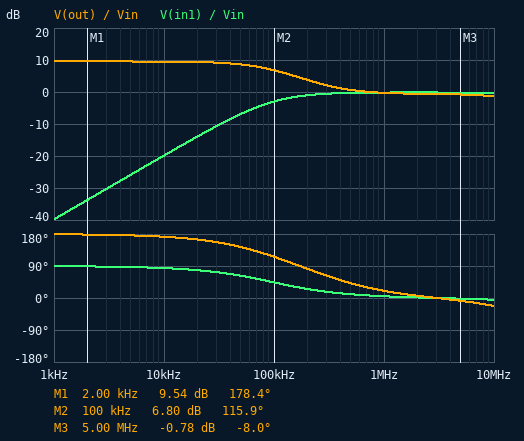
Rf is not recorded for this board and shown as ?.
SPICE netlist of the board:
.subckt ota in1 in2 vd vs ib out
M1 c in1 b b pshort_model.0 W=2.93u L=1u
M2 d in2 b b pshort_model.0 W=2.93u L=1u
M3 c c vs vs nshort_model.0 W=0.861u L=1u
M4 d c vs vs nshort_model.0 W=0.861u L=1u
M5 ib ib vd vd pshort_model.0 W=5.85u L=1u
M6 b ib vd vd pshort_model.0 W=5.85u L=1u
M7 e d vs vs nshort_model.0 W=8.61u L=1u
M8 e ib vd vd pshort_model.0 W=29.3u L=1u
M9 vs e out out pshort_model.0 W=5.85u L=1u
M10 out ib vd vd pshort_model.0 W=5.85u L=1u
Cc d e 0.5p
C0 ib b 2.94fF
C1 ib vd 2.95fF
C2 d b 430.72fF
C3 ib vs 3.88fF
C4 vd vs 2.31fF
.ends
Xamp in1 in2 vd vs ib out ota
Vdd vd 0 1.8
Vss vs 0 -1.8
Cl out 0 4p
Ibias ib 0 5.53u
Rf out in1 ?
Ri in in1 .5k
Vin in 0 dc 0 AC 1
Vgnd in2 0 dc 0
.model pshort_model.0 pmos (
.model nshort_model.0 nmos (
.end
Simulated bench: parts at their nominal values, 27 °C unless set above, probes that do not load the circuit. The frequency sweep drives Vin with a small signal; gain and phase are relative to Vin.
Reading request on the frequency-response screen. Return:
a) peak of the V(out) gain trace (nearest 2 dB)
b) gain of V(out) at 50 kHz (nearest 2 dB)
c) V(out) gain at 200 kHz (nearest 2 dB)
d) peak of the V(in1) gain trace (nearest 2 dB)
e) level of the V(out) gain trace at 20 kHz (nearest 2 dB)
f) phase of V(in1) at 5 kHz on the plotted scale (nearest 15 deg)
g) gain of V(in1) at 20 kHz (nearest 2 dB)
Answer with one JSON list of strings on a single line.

["10 dB", "8 dB", "4 dB", "0 dB", "10 dB", "90 deg", "-14 dB"]
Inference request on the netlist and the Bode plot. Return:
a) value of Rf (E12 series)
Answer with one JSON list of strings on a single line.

["1.5 kΩ"]
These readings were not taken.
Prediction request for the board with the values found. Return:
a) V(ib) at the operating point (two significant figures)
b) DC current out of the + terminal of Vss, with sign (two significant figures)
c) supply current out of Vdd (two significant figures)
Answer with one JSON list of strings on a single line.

["1.5 V", "-39 µA", "44 µA"]
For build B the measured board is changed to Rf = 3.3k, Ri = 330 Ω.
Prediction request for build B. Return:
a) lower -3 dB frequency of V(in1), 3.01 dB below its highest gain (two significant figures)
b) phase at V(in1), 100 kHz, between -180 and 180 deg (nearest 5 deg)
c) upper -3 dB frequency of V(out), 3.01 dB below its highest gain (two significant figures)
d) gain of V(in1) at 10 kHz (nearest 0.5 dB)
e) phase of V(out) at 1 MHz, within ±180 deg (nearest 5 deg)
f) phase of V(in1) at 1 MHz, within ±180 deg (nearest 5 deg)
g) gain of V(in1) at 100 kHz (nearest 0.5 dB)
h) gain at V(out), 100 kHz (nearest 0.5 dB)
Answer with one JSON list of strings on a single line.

["60 kHz", "30 deg", "61 kHz", "-16.0 dB", "35 deg", "5 deg", "-1.5 dB", "14.5 dB"]
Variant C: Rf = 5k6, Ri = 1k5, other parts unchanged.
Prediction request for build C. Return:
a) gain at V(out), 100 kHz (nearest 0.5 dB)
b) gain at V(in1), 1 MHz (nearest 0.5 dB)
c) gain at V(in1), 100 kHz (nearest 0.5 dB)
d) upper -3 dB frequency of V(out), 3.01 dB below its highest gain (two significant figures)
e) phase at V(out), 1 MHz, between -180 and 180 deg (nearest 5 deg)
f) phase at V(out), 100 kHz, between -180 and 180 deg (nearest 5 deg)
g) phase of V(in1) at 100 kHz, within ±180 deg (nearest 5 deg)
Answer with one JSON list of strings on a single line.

["11.0 dB", "-0.5 dB", "-9.0 dB", "270 kHz", "55 deg", "155 deg", "70 deg"]
